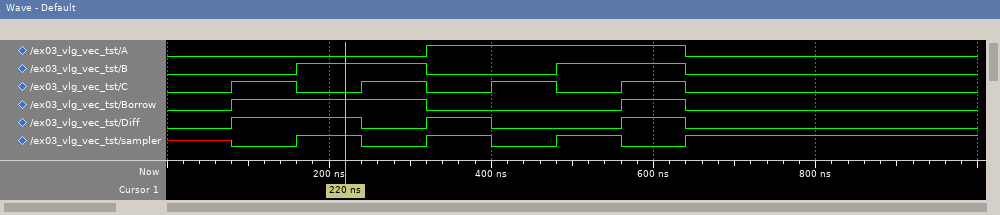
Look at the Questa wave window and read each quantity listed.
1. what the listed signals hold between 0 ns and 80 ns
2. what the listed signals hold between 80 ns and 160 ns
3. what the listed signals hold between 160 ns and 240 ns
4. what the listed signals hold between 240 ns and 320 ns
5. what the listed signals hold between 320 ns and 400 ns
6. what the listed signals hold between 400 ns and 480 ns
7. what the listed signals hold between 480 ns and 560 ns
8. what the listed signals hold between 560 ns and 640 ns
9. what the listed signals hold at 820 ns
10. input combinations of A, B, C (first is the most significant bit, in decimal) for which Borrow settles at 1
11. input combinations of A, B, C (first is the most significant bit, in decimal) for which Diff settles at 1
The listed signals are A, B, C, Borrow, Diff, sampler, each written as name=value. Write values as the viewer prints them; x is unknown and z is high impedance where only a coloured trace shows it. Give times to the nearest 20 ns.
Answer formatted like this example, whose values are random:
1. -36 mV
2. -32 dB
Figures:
1. A=0, B=0, C=0, Borrow=0, Diff=0, sampler=x
2. A=0, B=0, C=1, Borrow=1, Diff=1, sampler=0
3. A=0, B=1, C=0, Borrow=1, Diff=1, sampler=1
4. A=0, B=1, C=1, Borrow=1, Diff=0, sampler=0
5. A=1, B=0, C=0, Borrow=0, Diff=1, sampler=1
6. A=1, B=0, C=1, Borrow=0, Diff=0, sampler=0
7. A=1, B=1, C=0, Borrow=0, Diff=0, sampler=1
8. A=1, B=1, C=1, Borrow=1, Diff=1, sampler=0
9. A=0, B=0, C=0, Borrow=0, Diff=0, sampler=1
10. 1, 2, 3, 7
11. 1, 2, 4, 7
